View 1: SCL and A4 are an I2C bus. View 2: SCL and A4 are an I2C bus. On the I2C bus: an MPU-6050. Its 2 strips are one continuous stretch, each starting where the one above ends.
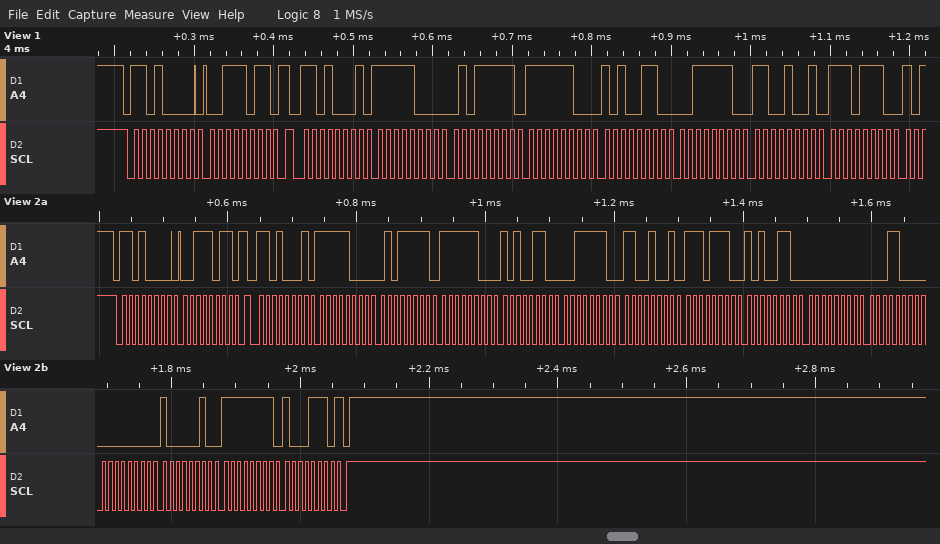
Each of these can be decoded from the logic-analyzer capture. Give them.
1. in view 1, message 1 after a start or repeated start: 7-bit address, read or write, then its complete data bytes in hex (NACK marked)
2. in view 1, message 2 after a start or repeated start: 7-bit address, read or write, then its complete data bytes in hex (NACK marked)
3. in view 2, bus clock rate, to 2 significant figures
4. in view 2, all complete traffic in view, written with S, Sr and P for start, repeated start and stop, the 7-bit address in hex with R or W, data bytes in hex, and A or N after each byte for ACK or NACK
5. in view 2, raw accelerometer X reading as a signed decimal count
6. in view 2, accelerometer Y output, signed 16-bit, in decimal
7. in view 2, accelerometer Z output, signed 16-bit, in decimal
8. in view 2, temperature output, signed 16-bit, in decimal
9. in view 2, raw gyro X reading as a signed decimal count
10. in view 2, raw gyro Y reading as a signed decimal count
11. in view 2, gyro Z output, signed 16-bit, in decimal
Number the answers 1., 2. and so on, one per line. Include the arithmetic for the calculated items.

1. 0x68 write: 3B
2. 0x68 read: F8 5F FC A6 3E C9 EE
3. 100 kHz
4. S 68W A 3B A Sr 68R A F8 A 5F A FC A A6 A 3E A C9 A EE A A6 A 00 A 18 A 00 A 82 A FF A 8E N P
5. 0xF85F = -1953
6. 0xFCA6 = -858
7. 0x3EC9 = 16073
8. 0xEEA6 = -4442
9. 0x0018 = 24
10. 0x0082 = 130
11. 0xFF8E = -114
